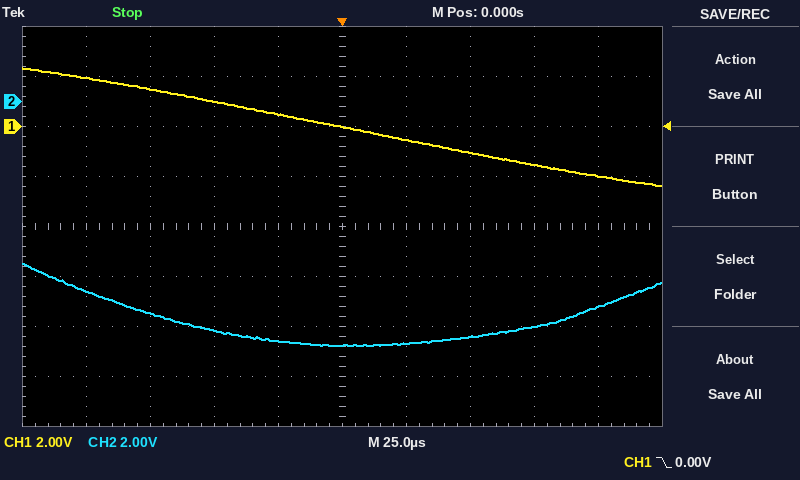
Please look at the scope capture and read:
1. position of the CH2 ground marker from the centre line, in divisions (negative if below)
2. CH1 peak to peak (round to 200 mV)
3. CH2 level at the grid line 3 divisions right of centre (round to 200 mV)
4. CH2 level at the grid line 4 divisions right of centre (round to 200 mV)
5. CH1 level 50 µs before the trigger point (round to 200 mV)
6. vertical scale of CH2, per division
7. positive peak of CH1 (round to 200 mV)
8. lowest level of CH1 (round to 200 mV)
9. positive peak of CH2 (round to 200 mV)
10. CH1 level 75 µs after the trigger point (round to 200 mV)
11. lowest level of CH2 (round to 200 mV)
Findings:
+2.5 div
4.8 V
-9.0 V
-8.2 V
1.0 V
2 V
2.4 V
-2.4 V
-6.4 V
-1.6 V
-9.8 V
